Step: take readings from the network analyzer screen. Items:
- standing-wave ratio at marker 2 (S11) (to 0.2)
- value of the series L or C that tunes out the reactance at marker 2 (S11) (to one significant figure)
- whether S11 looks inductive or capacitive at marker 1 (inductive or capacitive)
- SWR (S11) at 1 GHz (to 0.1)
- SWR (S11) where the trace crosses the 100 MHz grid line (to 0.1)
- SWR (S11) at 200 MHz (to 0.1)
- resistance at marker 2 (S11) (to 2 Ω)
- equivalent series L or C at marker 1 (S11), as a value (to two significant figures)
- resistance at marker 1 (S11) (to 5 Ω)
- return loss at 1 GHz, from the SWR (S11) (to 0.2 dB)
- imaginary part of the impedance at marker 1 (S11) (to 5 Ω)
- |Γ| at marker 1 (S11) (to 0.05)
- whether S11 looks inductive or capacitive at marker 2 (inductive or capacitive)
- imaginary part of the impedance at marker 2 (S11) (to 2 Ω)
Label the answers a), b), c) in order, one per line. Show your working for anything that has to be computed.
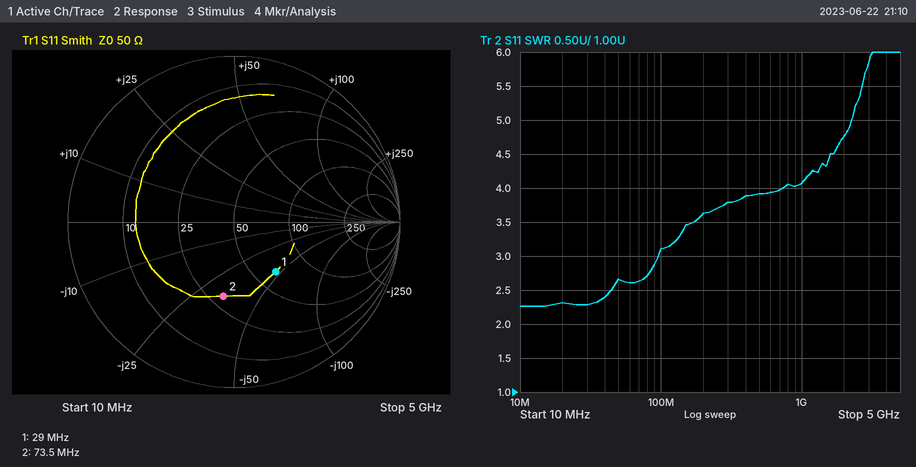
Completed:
a) 2.6
b) L = 34 Ω/(2π × 73.5 MHz) ≈ 73.6 nH, so 70 nH to one significant figure
c) capacitive
d) 4.1
e) 3.1
f) 3.6
g) 30 Ω
h) C = 1/(2π × 29 MHz × 45 Ω) ≈ 122 pF, so 120 pF to two significant figures
i) 65 Ω
j) −20 log10((4.1 − 1)/(4.1 + 1)) ≈ 4.32 dB, so 4.4 dB to the nearest 0.2 dB
k) -45 Ω
l) 0.40
m) capacitive
n) -34 Ω
